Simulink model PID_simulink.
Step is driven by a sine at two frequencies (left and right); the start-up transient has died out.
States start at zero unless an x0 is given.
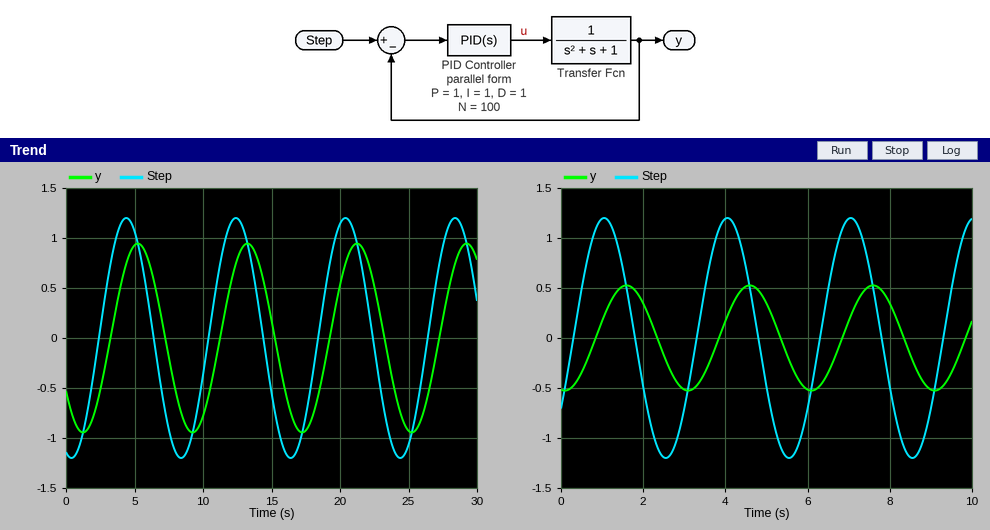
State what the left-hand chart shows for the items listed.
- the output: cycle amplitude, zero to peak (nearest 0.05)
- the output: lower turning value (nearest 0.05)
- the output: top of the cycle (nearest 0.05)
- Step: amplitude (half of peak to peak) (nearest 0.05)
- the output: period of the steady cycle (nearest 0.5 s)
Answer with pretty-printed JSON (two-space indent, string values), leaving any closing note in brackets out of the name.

{
  "the output: cycle amplitude, zero to peak": "0.95",
  "the output: lower turning value": "-0.95",
  "the output: top of the cycle": "0.95",
  "Step: amplitude (half of peak to peak)": "1.20",
  "the output: period of the steady cycle": "8.0 s"
}
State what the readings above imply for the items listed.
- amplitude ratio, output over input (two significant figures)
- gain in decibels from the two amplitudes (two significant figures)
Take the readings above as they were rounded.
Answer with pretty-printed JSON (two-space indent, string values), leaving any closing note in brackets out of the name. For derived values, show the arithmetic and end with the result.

{
  "amplitude ratio, output over input": "0.95 / 1.2 = 0.79",
  "gain in decibels from the two amplitudes": "20 log10(0.95 / 1.2) = -2.0 dB"
}
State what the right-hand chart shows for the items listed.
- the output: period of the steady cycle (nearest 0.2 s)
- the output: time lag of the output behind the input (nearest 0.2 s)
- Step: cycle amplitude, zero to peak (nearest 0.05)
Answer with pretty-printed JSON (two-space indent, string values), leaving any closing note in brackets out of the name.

{
  "the output: period of the steady cycle": "3.0 s",
  "the output: time lag of the output behind the input": "0.6 s",
  "Step: cycle amplitude, zero to peak": "1.20"
}
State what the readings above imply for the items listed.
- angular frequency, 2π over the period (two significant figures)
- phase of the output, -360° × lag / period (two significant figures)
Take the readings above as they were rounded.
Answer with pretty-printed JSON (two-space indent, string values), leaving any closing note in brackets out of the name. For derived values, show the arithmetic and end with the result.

{
  "angular frequency, 2π over the period": "2π / 3 = 2.1 rad/s",
  "phase of the output, -360° × lag / period": "-360 × 0.6 / 3 = -72°"
}
